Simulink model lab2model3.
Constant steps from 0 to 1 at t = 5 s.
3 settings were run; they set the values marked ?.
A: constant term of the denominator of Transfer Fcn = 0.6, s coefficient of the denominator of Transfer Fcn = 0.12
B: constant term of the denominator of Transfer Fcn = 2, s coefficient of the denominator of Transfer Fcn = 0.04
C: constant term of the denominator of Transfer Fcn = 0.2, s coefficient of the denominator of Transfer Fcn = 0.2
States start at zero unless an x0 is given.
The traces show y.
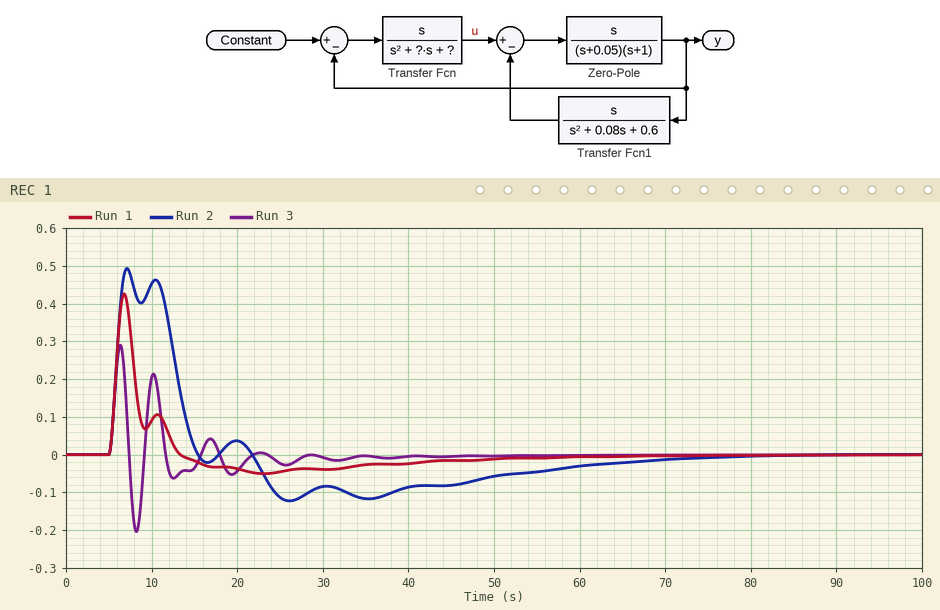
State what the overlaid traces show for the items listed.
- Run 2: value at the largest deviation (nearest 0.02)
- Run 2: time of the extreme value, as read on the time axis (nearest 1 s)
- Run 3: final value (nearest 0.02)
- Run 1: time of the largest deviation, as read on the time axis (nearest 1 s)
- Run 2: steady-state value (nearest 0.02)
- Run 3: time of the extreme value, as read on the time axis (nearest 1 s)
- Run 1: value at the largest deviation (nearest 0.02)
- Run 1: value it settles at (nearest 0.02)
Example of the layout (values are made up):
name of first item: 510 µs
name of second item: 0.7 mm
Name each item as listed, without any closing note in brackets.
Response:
Run 2: value at the largest deviation: 0.50
Run 2: time of the extreme value, as read on the time axis: 7 s
Run 3: final value: 0.00
Run 1: time of the largest deviation, as read on the time axis: 7 s
Run 2: steady-state value: 0.00
Run 3: time of the extreme value, as read on the time axis: 6 s
Run 1: value at the largest deviation: 0.42
Run 1: value it settles at: 0.00
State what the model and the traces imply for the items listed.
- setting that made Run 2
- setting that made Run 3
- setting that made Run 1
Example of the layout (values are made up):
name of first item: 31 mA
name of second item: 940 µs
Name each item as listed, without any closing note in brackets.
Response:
setting that made Run 2: C
setting that made Run 3: B
setting that made Run 1: A
